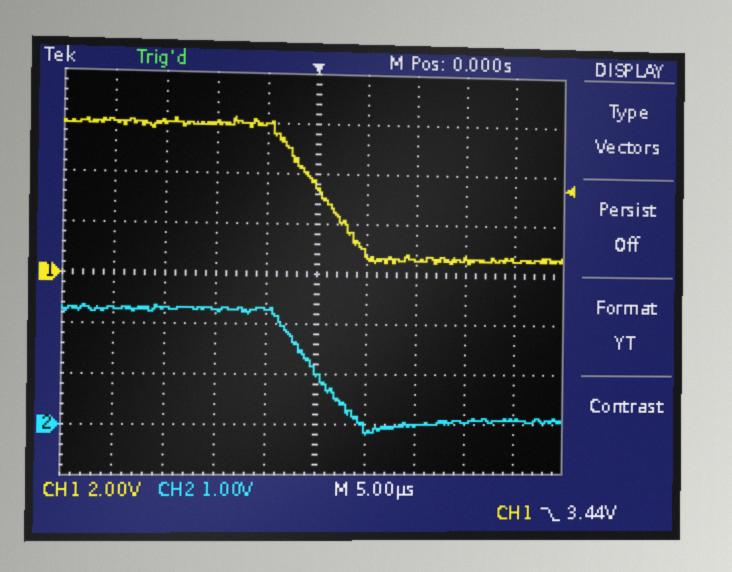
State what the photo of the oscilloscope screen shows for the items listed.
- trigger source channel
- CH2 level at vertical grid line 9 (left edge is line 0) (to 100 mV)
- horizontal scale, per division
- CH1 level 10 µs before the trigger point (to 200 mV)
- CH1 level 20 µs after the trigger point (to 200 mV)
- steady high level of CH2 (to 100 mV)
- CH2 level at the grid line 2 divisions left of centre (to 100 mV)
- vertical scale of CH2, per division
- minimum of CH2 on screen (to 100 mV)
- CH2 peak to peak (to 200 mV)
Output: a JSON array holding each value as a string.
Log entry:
["CH1", "100 mV", "5 µs", "6.0 V", "600 mV", "2.3 V", "2.3 V", "1 V", "-200 mV", "2.6 V"]
